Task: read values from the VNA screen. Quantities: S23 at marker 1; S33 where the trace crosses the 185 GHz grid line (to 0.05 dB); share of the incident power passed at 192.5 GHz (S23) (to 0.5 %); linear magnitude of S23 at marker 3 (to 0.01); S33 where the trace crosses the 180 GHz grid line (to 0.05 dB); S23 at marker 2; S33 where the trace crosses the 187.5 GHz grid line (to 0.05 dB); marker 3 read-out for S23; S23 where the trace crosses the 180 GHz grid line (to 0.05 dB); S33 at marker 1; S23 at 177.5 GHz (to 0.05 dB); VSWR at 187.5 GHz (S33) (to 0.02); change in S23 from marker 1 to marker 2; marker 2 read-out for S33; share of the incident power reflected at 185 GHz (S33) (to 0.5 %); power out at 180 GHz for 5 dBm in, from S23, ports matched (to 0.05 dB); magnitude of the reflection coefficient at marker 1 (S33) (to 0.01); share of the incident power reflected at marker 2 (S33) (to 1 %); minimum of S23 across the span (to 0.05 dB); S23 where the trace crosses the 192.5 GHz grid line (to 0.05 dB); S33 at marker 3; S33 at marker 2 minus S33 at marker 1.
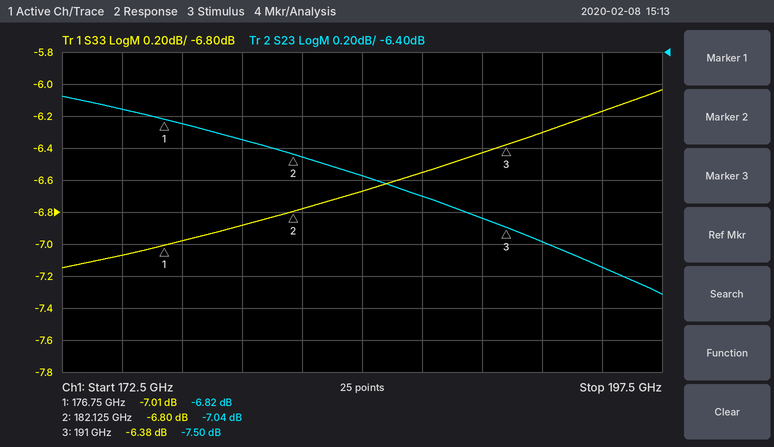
-6.82 dB
-6.65 dB
17.5 %
0.42
-6.90 dB
-7.04 dB
-6.55 dB
-7.50 dB
-6.95 dB
-7.01 dB
-6.85 dB
2.78
-0.22 dB
-6.80 dB
21.5 %
-1.95 dBm
0.45
21 %
-7.90 dB
-7.60 dB
-6.38 dB
0.21 dB
